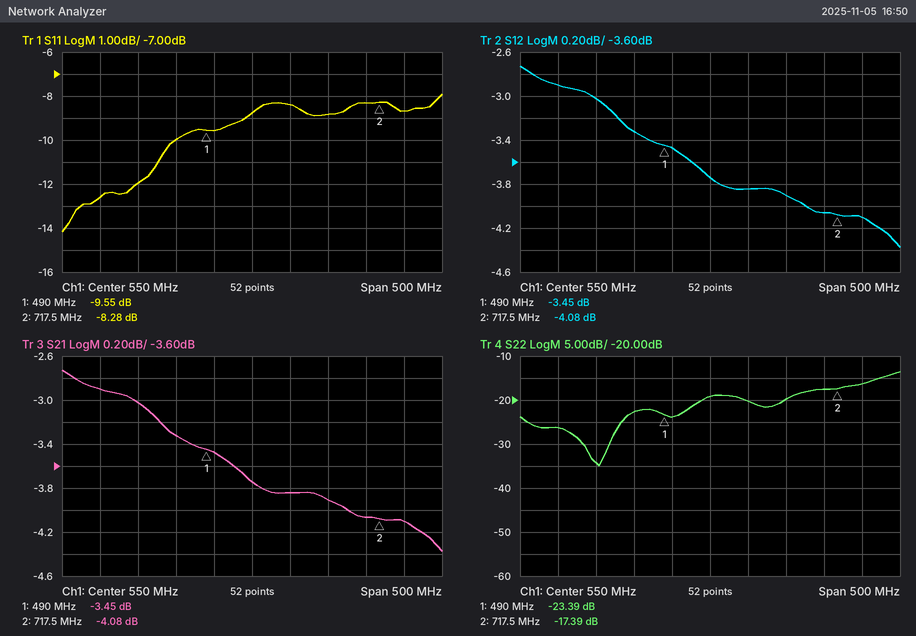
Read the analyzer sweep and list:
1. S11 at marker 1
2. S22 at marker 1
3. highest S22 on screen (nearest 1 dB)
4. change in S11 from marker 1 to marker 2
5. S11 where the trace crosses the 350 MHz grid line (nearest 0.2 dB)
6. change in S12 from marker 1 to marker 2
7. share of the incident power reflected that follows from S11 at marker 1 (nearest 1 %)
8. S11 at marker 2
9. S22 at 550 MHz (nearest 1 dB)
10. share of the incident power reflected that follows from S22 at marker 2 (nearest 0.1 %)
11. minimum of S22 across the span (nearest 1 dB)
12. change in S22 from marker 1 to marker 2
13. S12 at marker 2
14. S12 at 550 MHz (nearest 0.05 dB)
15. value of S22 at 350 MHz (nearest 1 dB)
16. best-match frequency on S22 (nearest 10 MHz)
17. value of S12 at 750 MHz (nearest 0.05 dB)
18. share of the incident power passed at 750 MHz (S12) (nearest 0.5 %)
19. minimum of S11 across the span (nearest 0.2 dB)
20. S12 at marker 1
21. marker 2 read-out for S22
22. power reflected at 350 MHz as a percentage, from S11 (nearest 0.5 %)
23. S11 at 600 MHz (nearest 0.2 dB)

-9.55 dB
-23.39 dB
-14 dB
1.27 dB
-12.6 dB
-0.63 dB
11 %
-8.28 dB
-19 dB
1.8 %
-35 dB
6.00 dB
-4.08 dB
-3.75 dB
-26 dB
400 MHz
-4.10 dB
39.0 %
-14.2 dB
-3.45 dB
-17.39 dB
5.5 %
-8.4 dB
